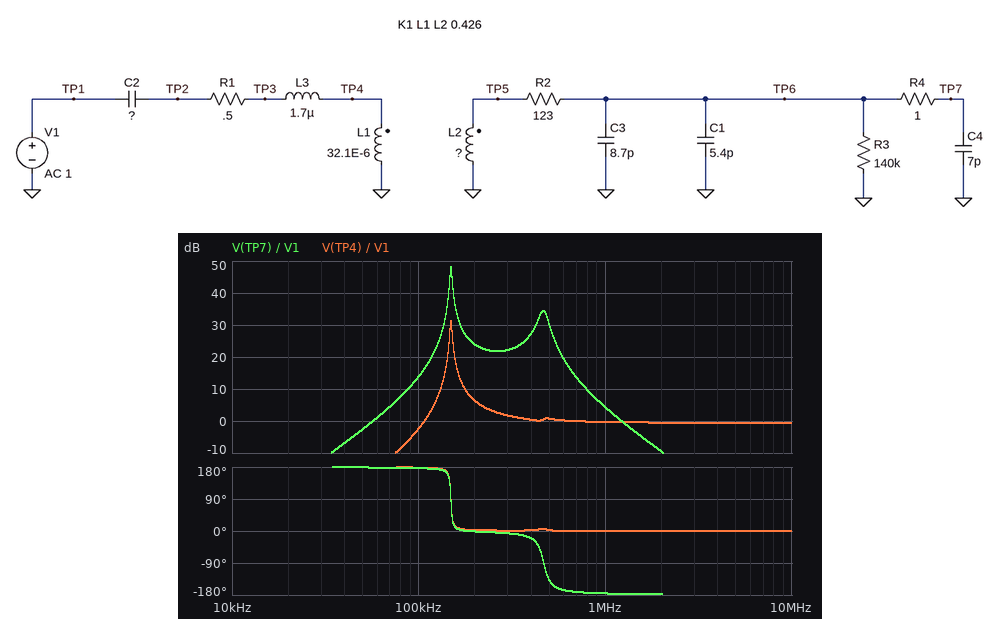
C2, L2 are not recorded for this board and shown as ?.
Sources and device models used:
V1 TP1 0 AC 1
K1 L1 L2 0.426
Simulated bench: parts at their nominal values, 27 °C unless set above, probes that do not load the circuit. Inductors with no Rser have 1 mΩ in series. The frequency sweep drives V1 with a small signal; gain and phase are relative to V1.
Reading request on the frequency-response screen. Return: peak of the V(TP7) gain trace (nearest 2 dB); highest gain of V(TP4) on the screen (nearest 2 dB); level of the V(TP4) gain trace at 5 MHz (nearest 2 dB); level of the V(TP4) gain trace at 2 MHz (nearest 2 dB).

48 dB
32 dB
0 dB
0 dB
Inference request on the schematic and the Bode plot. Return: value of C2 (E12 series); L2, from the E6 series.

33 nF
6.8 mH
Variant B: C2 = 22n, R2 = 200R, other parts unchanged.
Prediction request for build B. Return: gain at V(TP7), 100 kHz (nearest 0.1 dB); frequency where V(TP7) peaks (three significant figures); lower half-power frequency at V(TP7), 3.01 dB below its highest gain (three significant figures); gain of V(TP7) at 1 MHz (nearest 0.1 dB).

8.3 dB
181 kHz
179 kHz
4.4 dB
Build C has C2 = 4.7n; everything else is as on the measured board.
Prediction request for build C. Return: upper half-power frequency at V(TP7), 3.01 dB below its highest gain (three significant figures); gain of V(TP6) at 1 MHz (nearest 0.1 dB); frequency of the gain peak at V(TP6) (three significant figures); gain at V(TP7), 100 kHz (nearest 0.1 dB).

551 kHz
6.0 dB
534 kHz
-7.6 dB
